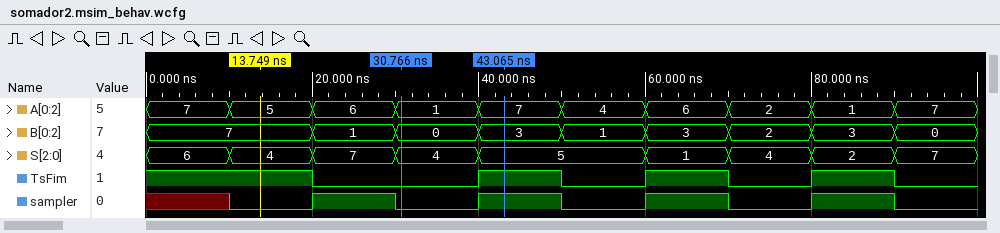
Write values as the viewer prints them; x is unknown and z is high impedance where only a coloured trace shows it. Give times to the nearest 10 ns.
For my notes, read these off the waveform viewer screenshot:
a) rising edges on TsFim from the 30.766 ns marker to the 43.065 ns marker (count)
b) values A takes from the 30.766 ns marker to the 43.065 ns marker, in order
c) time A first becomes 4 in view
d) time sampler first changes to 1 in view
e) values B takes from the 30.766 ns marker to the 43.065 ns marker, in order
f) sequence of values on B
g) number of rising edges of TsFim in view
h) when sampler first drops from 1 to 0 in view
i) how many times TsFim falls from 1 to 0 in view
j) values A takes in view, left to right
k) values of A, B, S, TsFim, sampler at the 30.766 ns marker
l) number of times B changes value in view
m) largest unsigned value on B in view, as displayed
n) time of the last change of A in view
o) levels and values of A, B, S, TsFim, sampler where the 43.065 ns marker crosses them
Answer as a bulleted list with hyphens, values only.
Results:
- 1
- 1, 7
- 50 ns
- 20 ns
- 0, 3
- 7, 1, 0, 3, 1, 3, 2, 3, 0
- 3
- 30 ns
- 4
- 7, 5, 6, 1, 7, 4, 6, 2, 1, 7
- A=1, B=0, S=4, TsFim=0, sampler=0
- 8
- 7
- 90 ns
- A=7, B=3, S=5, TsFim=1, sampler=1
